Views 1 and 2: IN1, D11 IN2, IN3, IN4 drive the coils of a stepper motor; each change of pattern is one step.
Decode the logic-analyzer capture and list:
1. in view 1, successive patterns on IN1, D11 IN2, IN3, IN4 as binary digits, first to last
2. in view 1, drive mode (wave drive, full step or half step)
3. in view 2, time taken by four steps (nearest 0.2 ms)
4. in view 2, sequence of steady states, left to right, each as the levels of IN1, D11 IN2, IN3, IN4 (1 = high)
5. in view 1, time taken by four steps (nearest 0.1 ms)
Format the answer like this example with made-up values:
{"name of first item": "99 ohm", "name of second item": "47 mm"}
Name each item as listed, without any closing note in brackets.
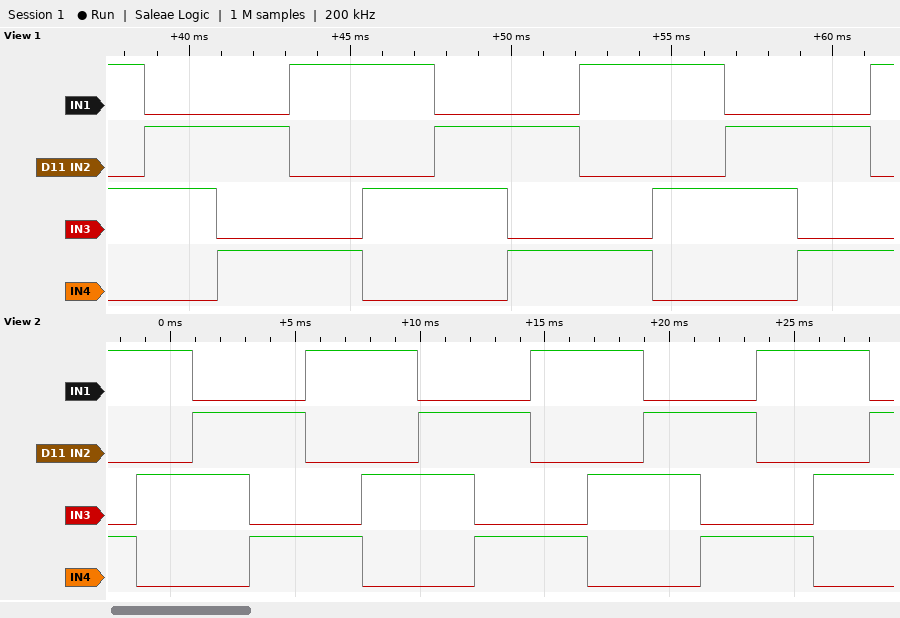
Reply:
{"in view 1, successive patterns on IN1, D11 IN2, IN3, IN4 as binary digits, first to last": "1010 0110 0101 1001 1010 0110 0101 1001 1010 0110 0101 1001", "in view 1, drive mode": "full step", "in view 2, time taken by four steps": "9.0 ms", "in view 2, sequence of steady states, left to right, each as the levels of IN1, D11 IN2, IN3, IN4": "1001 1010 0110 0101 1001 1010 0110 0101 1001 1010 0110 0101 1001 1010 0110", "in view 1, time taken by four steps": "9.0 ms"}
